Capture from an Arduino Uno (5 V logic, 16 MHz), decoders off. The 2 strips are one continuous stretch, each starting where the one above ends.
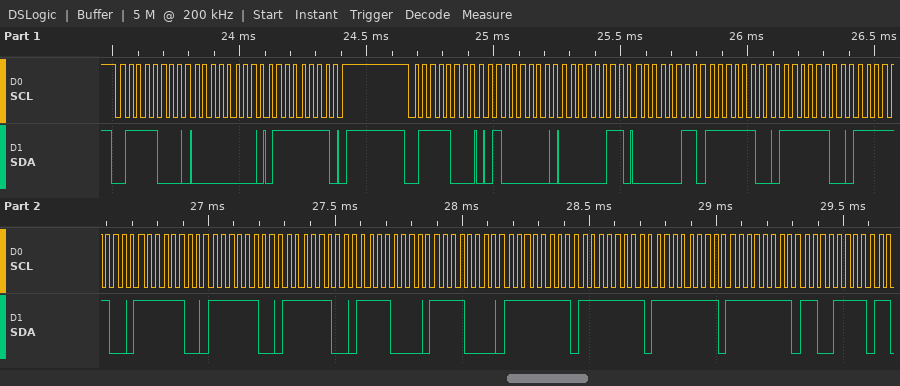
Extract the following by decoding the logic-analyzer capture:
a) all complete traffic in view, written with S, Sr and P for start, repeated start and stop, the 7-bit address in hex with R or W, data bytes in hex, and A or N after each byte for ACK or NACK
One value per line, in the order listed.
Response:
S 3CW A 00 A 7F A P S 3CW A 40 A 03 A 03 A FC A FC A FC A FC A FC A FC A F0 A F0 A FF A FF A FF A FF A CF A
